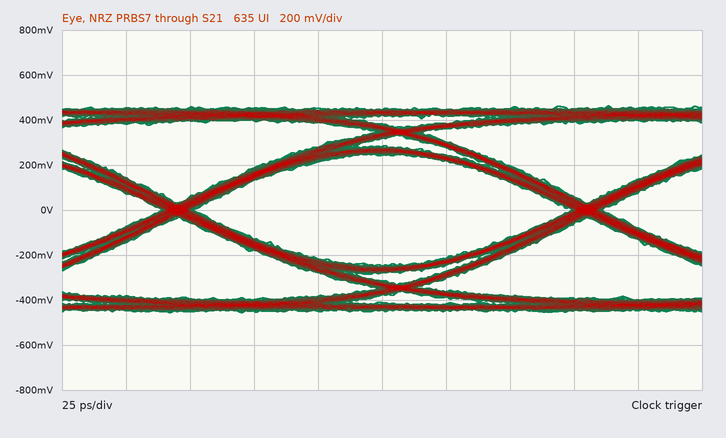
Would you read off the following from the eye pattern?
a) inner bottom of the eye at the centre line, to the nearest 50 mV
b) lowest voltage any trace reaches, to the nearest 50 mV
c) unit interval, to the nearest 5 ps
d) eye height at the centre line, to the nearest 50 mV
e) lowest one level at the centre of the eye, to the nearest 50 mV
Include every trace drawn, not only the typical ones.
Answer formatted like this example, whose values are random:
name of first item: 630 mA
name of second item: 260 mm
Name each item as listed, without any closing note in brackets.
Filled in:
inner bottom of the eye at the centre line, to the nearest 50 mV: -250 mV
lowest voltage any trace reaches, to the nearest 50 mV: -450 mV
unit interval, to the nearest 5 ps: 160 ps
eye height at the centre line, to the nearest 50 mV: 500 mV
lowest one level at the centre of the eye, to the nearest 50 mV: 250 mV
